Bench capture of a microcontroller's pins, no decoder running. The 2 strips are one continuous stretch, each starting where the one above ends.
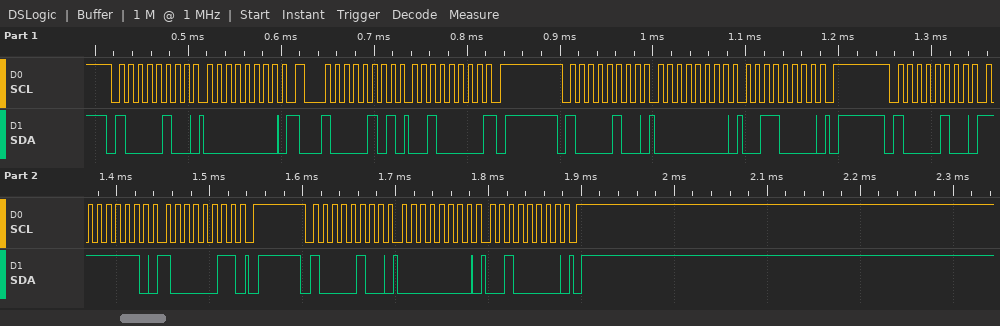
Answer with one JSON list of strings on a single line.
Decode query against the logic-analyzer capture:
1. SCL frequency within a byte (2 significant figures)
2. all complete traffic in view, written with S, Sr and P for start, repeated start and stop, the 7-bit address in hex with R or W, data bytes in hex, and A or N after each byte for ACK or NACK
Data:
["100 kHz", "S 42W A 00 A Sr 42R A 20 N P S 42W A 00 A 30 A P S 42W A FE A 83 A P S 42W A 00 A 20 A P"]
